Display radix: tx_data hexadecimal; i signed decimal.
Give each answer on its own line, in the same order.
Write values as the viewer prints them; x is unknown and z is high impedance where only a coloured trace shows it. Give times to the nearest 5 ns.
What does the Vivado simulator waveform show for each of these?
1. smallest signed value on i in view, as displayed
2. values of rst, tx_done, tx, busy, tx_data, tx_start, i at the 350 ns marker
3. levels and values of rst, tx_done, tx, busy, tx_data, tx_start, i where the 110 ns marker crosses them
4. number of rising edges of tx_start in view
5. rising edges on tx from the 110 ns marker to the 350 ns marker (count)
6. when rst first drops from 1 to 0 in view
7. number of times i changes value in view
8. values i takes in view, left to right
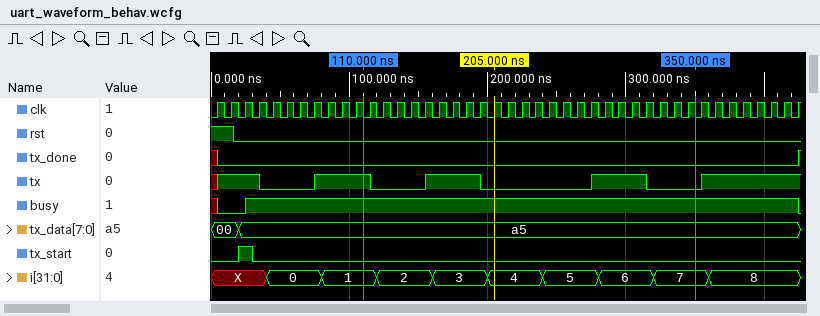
0
rst=0, tx_done=0, tx=0, busy=1, tx_data=a5, tx_start=0, i=7
rst=0, tx_done=0, tx=1, busy=1, tx_data=a5, tx_start=0, i=1
1
2
15 ns
9
X, 0, 1, 2, 3, 4, 5, 6, 7, 8
